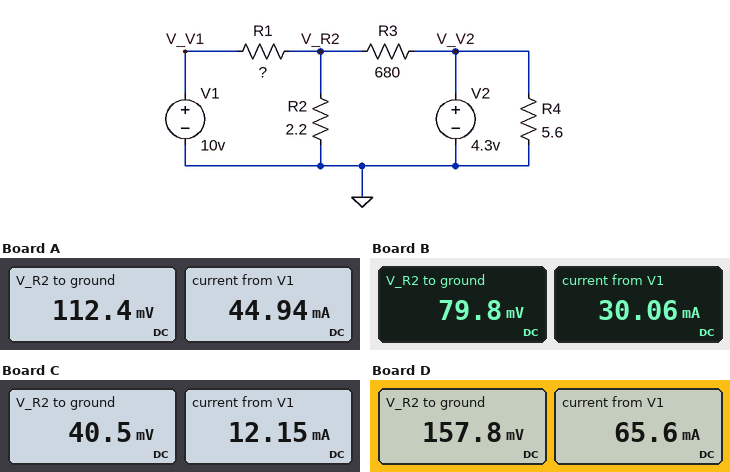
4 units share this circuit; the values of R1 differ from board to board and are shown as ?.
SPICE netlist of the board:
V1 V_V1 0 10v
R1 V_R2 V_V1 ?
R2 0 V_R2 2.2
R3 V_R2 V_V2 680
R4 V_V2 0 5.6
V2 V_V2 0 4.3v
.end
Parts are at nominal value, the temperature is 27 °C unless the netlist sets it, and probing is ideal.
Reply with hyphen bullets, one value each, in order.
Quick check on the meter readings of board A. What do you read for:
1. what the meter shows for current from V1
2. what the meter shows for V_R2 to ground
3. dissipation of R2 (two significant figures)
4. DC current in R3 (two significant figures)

- 44.94 mA
- 112.4 mV
- 5.7 mW
- 6.2 mA
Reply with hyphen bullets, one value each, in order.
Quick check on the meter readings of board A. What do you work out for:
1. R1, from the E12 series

- 220 Ω
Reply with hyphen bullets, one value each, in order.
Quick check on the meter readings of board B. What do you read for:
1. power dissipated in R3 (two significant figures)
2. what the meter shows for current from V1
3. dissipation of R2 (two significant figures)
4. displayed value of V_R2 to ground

- 26 mW
- 30.06 mA
- 2.9 mW
- 79.8 mV
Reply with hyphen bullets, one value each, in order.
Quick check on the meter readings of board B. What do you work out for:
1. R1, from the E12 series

- 330 Ω
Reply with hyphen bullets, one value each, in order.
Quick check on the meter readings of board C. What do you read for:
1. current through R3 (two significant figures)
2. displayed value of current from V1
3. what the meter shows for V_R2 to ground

- 6.3 mA
- 12.15 mA
- 40.5 mV
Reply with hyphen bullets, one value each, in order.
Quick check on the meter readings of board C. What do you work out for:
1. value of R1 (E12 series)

- 820 Ω
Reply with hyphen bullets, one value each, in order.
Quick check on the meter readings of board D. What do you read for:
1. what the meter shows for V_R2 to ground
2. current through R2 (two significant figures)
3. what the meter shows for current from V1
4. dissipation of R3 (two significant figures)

- 157.8 mV
- 72 mA
- 65.6 mA
- 25 mW
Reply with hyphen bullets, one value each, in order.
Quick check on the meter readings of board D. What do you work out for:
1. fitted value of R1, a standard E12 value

- 150 Ω
